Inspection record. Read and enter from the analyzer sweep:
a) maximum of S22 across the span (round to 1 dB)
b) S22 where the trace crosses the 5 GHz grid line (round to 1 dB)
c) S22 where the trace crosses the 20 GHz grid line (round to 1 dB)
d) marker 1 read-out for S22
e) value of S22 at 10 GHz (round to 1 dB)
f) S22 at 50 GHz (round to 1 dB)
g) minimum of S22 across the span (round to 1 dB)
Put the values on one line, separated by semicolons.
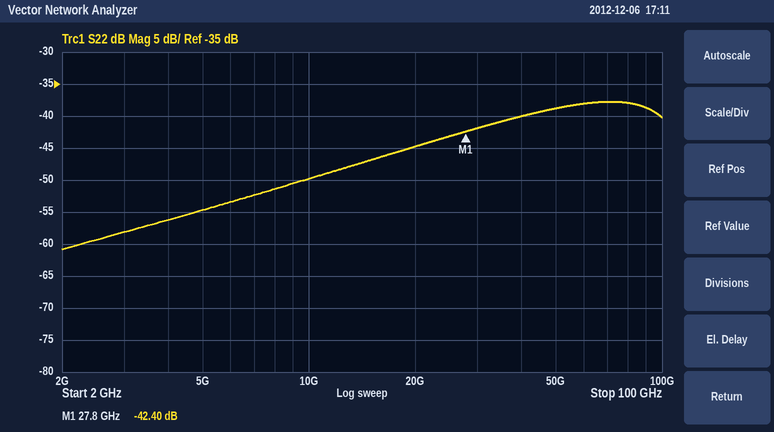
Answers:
-38 dB; -55 dB; -45 dB; -42.40 dB; -50 dB; -39 dB; -61 dB
